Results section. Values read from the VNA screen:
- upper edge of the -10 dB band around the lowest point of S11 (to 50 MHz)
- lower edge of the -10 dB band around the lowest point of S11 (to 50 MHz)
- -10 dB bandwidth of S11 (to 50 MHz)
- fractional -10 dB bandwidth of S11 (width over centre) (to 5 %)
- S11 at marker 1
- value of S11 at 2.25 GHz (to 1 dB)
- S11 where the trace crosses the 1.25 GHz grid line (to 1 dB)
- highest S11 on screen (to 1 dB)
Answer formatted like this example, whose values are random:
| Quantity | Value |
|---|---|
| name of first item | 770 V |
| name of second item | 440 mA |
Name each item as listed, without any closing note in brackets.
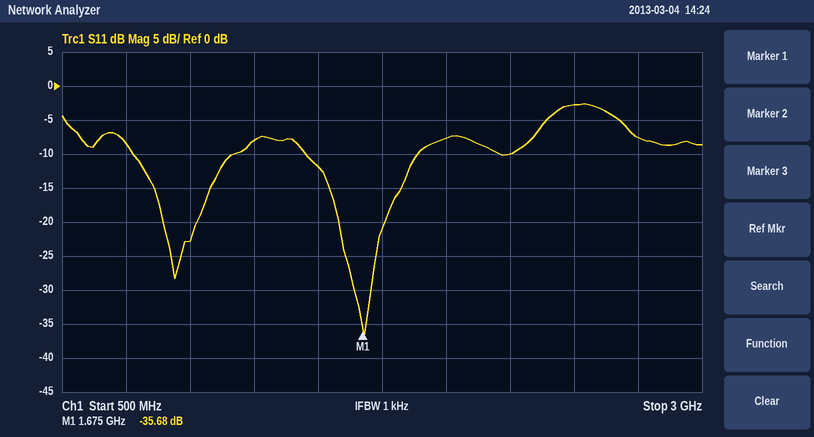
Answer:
| Quantity | Value |
|---|---|
| upper edge of the -10 dB band around the lowest point of S11 | 1.90 GHz |
| lower edge of the -10 dB band around the lowest point of S11 | 1.45 GHz |
| -10 dB bandwidth of S11 | 450 MHz |
| fractional -10 dB bandwidth of S11 (width over centre) | 25 % |
| S11 at marker 1 | -35.68 dB |
| value of S11 at 2.25 GHz | -10 dB |
| S11 where the trace crosses the 1.25 GHz grid line | -8 dB |
| highest S11 on screen | -3 dB |
